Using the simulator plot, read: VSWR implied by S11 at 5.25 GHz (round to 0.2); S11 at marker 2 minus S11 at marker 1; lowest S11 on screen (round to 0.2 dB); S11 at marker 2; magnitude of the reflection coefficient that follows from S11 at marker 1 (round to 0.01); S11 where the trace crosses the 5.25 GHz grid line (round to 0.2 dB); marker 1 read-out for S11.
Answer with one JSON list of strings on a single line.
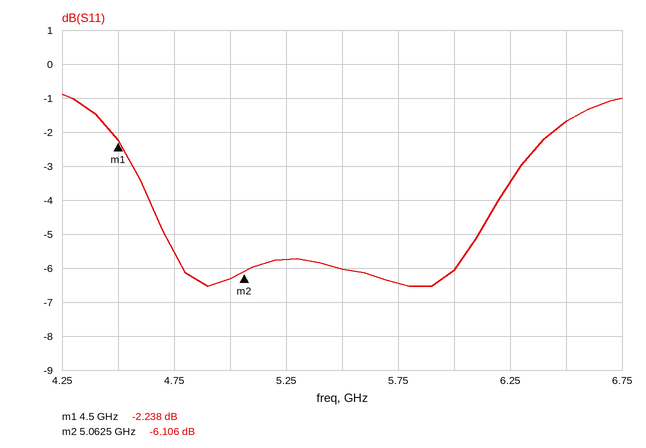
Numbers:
["3.2", "-3.868 dB", "-6.6 dB", "-6.106 dB", "0.77", "-5.8 dB", "-2.238 dB"]
